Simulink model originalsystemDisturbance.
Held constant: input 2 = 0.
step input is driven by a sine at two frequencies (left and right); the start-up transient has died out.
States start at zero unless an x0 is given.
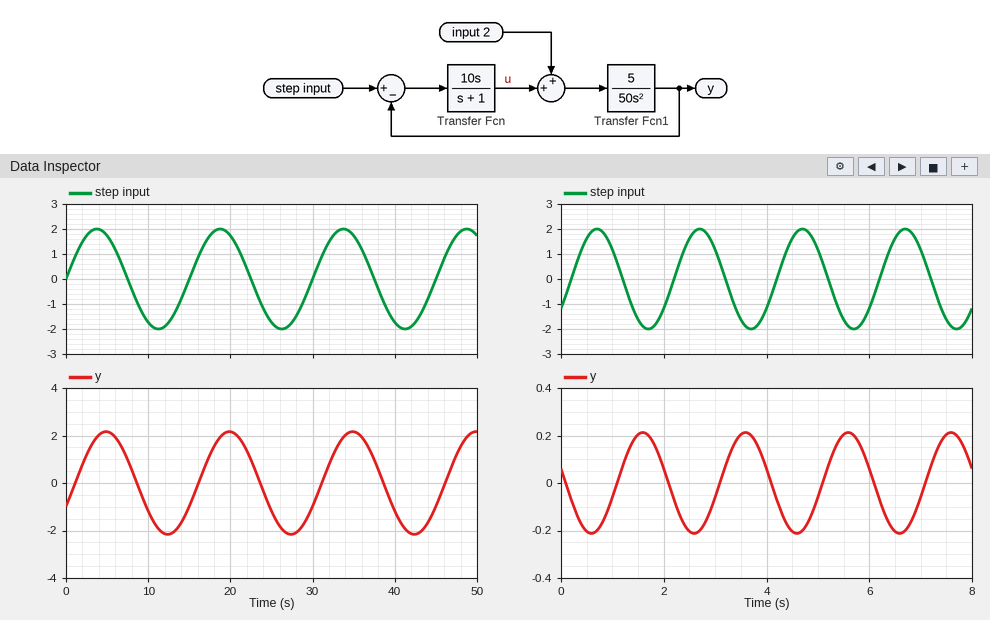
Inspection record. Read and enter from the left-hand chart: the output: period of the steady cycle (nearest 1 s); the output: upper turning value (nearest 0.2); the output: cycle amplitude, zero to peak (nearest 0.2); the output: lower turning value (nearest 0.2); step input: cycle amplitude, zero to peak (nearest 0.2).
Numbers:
15 s
2.2
2.2
-2.2
2.0
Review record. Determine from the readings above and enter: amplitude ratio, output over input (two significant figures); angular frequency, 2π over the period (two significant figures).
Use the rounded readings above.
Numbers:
1.1
0.42 rad/s
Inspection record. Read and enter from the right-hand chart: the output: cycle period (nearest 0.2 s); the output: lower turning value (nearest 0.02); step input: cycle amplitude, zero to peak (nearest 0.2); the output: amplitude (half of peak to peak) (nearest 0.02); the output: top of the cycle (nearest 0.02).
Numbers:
2.0 s
-0.22
2.0
0.22
0.22
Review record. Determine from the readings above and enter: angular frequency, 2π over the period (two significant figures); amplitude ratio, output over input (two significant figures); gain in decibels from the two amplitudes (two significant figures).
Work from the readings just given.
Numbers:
3.1 rad/s
0.11
-19 dB
